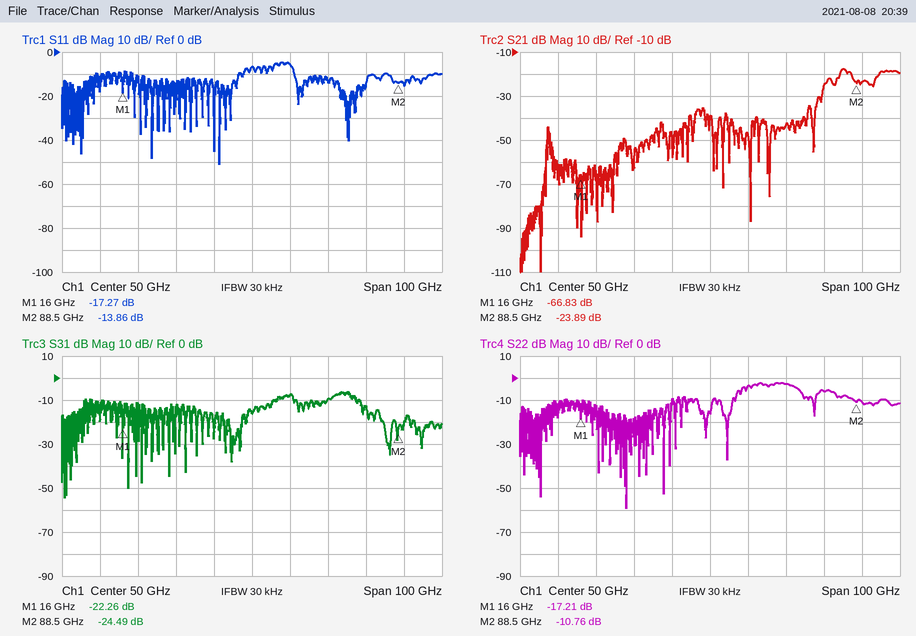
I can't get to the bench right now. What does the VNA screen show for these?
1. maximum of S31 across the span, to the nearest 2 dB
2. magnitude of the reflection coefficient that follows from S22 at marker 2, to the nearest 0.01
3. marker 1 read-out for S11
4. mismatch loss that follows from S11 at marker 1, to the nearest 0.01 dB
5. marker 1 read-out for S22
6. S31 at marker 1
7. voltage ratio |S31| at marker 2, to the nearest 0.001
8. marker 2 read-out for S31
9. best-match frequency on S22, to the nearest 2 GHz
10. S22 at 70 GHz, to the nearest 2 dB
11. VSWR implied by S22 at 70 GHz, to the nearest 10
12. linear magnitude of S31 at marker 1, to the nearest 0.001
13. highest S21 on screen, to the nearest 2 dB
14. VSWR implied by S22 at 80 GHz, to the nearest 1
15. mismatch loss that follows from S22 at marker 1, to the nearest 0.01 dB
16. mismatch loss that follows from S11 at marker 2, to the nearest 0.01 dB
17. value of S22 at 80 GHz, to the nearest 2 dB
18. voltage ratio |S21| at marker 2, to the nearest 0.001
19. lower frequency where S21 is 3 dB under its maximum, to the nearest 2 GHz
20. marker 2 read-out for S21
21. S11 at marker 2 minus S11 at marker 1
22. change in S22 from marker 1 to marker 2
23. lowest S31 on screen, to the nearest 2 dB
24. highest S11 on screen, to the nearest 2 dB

-6 dB
0.29
-17.27 dB
0.08 dB
-17.21 dB
-22.26 dB
0.060
-24.49 dB
28 GHz
-2 dB
10
0.077
-18 dB
3
0.08 dB
0.18 dB
-6 dB
0.064
84 GHz
-23.89 dB
3.41 dB
6.45 dB
-54 dB
-4 dB
